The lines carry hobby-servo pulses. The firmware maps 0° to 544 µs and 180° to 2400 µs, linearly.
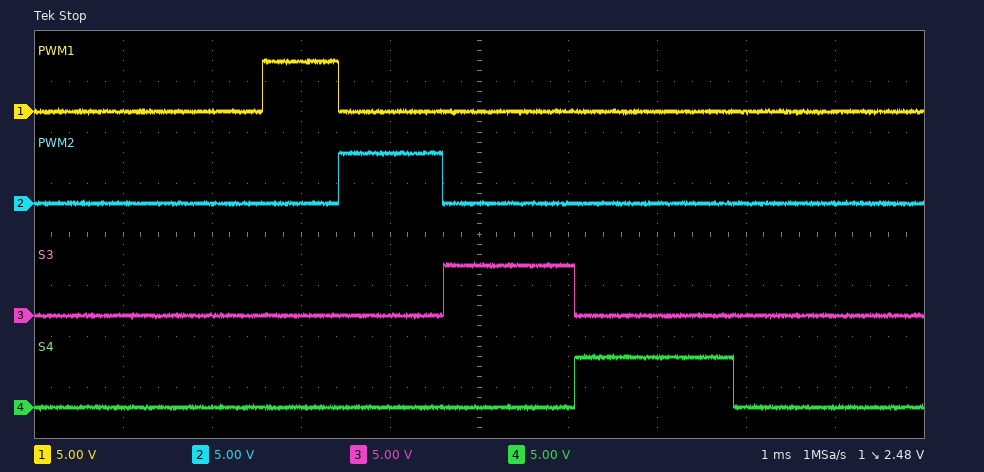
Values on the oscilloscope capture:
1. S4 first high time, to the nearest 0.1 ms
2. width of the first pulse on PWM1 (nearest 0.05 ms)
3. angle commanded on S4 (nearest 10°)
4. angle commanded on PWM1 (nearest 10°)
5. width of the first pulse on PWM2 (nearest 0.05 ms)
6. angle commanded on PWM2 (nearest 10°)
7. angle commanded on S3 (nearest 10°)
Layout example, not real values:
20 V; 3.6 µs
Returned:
1.8 ms; 0.85 ms; 120°; 30°; 1.15 ms; 60°; 90°
